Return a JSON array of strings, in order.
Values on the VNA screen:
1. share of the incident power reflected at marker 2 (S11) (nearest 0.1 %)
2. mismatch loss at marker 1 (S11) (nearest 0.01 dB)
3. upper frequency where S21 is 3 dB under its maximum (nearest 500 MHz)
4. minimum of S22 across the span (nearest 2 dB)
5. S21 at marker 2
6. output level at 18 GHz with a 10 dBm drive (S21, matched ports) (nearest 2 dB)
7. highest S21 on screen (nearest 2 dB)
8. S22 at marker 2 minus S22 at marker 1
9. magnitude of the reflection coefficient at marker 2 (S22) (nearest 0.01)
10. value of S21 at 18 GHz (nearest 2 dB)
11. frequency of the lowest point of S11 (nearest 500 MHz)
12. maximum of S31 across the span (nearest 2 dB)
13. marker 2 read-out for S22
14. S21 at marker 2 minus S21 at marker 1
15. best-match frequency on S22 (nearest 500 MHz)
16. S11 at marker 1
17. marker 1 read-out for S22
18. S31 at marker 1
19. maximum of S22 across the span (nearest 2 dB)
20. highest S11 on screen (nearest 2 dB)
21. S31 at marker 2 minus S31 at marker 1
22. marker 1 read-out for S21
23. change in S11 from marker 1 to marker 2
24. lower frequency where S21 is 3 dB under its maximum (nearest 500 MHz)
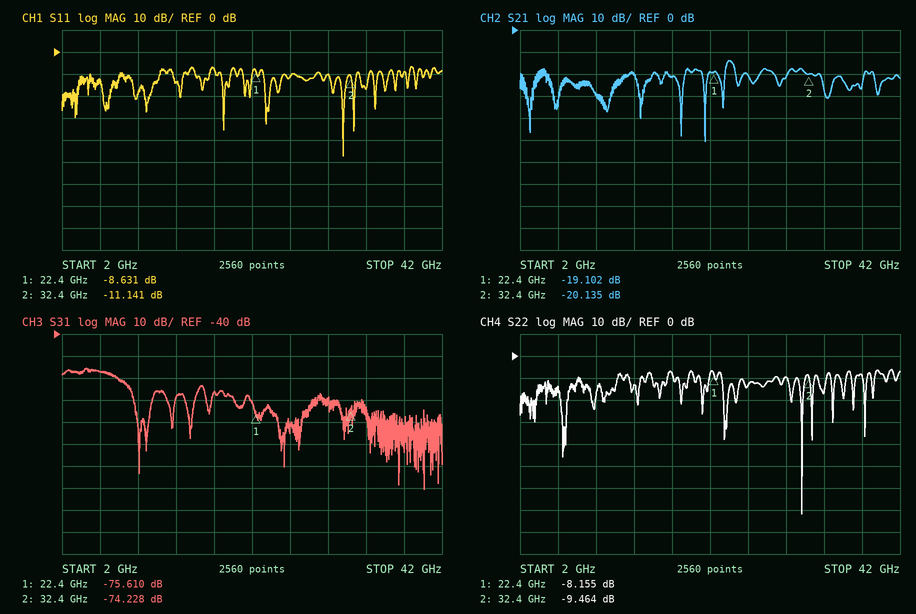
["7.7 %", "0.64 dB", "24.5 GHz", "-72 dB", "-20.135 dB", "-12 dBm", "-14 dB", "-1.309 dB", "0.34", "-22 dB", "31.5 GHz", "-56 dB", "-9.464 dB", "-1.033 dB", "31.5 GHz", "-8.631 dB", "-8.155 dB", "-75.610 dB", "-6 dB", "-6 dB", "1.382 dB", "-19.102 dB", "-2.510 dB", "23.5 GHz"]
